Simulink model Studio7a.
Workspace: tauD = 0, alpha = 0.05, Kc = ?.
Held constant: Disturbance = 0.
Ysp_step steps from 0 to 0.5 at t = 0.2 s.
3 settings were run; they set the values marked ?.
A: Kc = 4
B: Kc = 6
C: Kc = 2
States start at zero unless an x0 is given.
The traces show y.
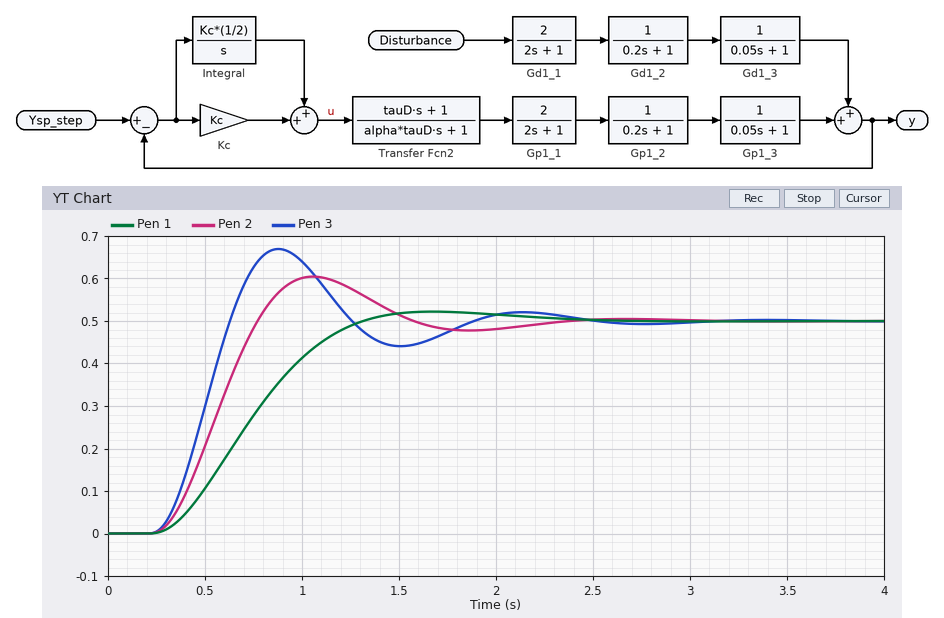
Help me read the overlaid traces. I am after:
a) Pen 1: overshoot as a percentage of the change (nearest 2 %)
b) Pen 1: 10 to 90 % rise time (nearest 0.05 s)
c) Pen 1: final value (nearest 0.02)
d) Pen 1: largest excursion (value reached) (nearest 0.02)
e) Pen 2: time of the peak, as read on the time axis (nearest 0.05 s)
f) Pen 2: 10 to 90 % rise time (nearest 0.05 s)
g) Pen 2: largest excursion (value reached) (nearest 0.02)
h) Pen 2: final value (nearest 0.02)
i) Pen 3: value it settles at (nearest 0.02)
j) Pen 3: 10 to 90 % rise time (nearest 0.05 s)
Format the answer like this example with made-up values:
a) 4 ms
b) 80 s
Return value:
a) 4 %
b) 0.70 s
c) 0.50
d) 0.52
e) 1.05 s
f) 0.35 s
g) 0.60
h) 0.50
i) 0.50
j) 0.25 s
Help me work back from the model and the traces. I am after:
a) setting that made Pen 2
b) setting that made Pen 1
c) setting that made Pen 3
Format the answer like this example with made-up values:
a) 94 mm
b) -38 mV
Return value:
a) A
b) C
c) B
